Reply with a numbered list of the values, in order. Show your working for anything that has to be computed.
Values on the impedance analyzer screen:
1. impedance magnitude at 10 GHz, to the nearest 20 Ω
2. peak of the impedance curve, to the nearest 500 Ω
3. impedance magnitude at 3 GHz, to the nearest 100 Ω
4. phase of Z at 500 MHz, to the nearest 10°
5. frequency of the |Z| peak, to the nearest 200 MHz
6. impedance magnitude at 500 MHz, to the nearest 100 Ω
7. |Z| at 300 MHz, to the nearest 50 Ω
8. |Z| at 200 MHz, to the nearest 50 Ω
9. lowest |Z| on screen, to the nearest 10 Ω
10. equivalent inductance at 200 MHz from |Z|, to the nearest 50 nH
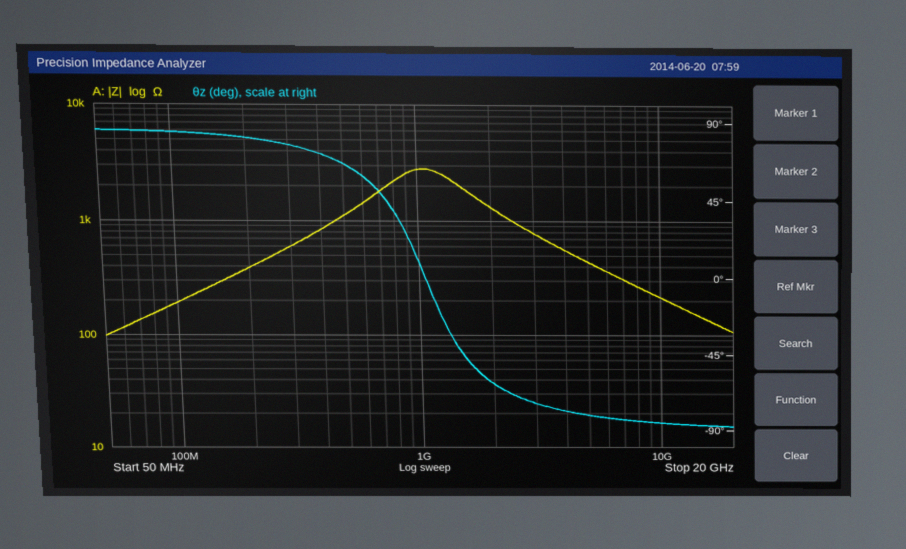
1. 220 Ω
2. 3.0 kΩ
3. 800 Ω
4. 70°
5. 1.0 GHz
6. 1.1 kΩ
7. 600 Ω
8. 400 Ω
9. 100 Ω
10. L = 400 Ω/(2π × 200 MHz) ≈ 318 nH, so 300 nH to the nearest 50 nH
